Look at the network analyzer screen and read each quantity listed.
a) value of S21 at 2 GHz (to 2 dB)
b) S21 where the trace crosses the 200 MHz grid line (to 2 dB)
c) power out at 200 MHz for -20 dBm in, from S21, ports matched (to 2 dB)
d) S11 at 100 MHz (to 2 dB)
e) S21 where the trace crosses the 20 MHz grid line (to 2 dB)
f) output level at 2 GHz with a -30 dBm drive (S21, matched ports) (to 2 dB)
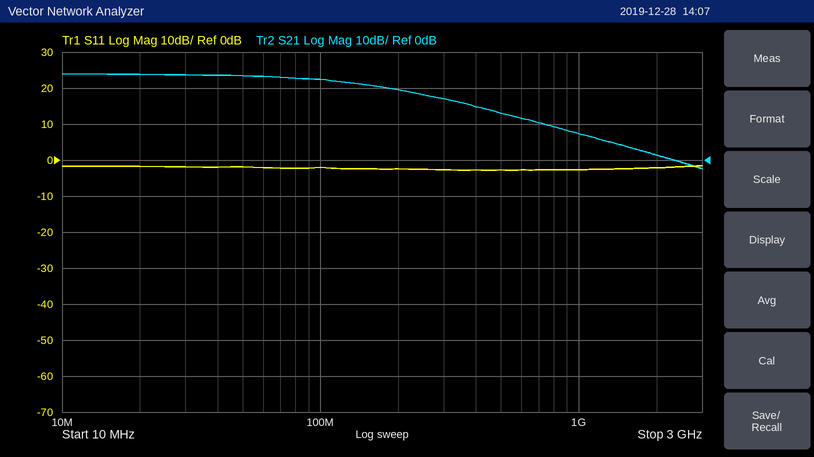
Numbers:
2 dB
20 dB
0 dBm
-2 dB
24 dB
-28 dBm
